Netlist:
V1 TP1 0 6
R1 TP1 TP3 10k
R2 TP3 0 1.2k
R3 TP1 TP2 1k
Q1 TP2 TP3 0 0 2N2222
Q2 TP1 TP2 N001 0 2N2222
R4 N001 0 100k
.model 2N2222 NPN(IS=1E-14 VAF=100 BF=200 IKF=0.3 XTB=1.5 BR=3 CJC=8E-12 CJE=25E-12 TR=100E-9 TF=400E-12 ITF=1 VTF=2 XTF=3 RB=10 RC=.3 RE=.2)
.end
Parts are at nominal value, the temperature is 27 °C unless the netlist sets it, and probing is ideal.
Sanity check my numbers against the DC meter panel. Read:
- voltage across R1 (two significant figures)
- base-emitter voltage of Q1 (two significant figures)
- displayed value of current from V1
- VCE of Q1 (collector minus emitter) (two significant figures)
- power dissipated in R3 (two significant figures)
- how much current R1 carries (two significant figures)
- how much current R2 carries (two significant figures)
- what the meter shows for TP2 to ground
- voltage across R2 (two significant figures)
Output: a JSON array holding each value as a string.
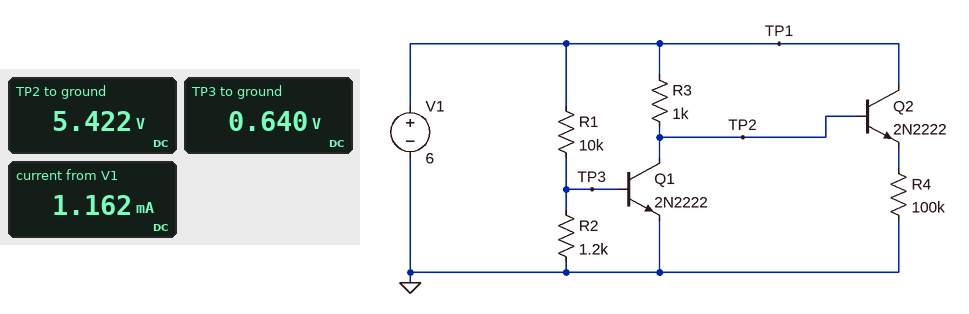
["5.4 V", "640 mV", "1.162 mA", "5.4 V", "330 µW", "540 µA", "530 µA", "5.422 V", "640 mV"]
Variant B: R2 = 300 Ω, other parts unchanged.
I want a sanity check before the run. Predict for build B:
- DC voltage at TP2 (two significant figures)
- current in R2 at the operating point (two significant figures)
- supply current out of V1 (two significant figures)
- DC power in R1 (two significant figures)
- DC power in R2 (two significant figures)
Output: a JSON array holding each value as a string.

["6.0 V", "580 µA", "640 µA", "3.4 mW", "100 µW"]
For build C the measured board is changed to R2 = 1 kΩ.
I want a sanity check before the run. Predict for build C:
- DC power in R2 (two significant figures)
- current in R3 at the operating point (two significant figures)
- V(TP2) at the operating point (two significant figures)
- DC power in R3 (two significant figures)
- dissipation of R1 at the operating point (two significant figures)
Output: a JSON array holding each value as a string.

["300 µW", "15 µA", "6.0 V", "240 nW", "3.0 mW"]
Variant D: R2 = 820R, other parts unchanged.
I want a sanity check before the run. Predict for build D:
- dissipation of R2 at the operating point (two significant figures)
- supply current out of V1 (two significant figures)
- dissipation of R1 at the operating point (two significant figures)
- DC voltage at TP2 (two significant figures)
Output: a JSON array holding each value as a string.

["250 µW", "610 µA", "3.1 mW", "6.0 V"]
